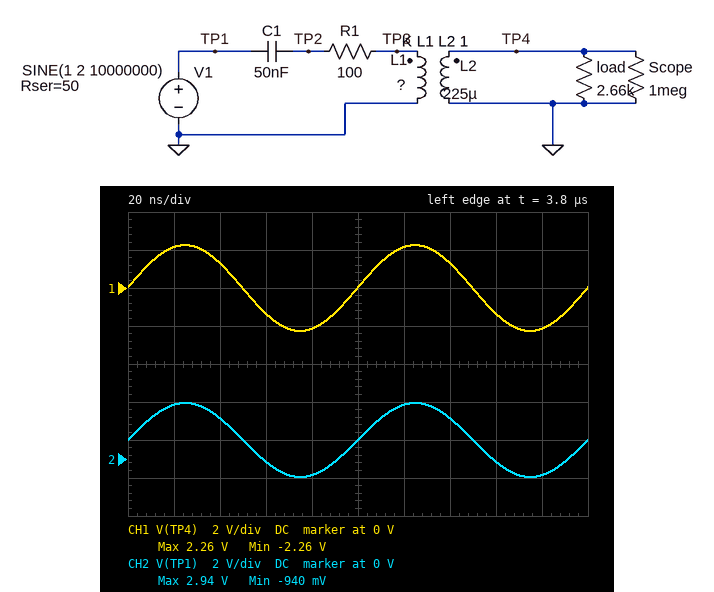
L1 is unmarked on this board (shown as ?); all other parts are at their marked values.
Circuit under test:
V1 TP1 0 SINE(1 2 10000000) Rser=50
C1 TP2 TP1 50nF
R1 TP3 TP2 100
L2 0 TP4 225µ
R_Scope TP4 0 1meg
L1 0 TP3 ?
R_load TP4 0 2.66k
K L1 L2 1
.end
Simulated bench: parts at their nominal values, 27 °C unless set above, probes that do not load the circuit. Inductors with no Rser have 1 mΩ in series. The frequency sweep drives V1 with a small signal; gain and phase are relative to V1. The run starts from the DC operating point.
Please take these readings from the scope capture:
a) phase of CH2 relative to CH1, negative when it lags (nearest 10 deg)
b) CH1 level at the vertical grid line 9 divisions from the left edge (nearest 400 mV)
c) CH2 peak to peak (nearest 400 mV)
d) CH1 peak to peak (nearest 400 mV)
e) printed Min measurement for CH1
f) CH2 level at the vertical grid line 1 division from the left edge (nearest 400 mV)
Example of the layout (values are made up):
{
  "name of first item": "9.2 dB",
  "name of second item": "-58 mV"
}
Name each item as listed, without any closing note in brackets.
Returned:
{
  "phase of CH2 relative to CH1, negative when it lags": "0 deg",
  "CH1 level at the vertical grid line 9 divisions from the left edge": "-2.0 V",
  "CH2 peak to peak": "4.0 V",
  "CH1 peak to peak": "4.4 V",
  "printed Min measurement for CH1": "-2.26 V",
  "CH2 level at the vertical grid line 1 division from the left edge": "2.8 V"
}
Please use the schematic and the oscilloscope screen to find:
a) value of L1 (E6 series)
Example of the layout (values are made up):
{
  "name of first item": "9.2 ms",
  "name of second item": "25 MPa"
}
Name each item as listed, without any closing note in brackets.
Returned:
{
  "value of L1": "150 µH"
}
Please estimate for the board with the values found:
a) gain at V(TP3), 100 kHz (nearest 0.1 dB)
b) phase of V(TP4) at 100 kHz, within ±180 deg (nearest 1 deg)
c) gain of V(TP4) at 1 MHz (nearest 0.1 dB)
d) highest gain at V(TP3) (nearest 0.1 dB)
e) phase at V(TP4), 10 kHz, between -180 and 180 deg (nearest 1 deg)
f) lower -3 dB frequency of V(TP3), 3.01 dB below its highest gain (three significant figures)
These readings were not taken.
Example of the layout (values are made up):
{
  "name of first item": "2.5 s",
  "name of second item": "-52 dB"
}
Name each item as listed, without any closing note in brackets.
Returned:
{
  "gain at V(TP3), 100 kHz": "-5.0 dB",
  "phase of V(TP4) at 100 kHz, within ±180 deg": "65 deg",
  "gain of V(TP4) at 1 MHz": "1.0 dB",
  "highest gain at V(TP3)": "-0.7 dB",
  "phase at V(TP4), 10 kHz, between -180 and 180 deg": "154 deg",
  "lower -3 dB frequency of V(TP3), 3.01 dB below its highest gain": "128 kHz"
}
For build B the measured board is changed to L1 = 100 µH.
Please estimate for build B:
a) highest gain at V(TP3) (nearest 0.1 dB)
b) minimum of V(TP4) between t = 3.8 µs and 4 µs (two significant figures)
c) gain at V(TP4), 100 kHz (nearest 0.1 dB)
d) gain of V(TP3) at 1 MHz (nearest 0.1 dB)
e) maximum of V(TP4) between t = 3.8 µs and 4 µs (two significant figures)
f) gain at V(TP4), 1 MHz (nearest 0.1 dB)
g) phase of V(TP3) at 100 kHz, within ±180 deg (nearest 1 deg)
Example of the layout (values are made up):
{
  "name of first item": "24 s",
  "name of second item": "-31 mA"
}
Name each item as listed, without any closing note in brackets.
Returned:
{
  "highest gain at V(TP3)": "-1.0 dB",
  "minimum of V(TP4) between t = 3.8 µs and 4 µs": "-2.7 V",
  "gain at V(TP4), 100 kHz": "-4.4 dB",
  "gain of V(TP3) at 1 MHz": "-1.2 dB",
  "maximum of V(TP4) between t = 3.8 µs and 4 µs": "2.7 V",
  "gain at V(TP4), 1 MHz": "2.3 dB",
  "phase of V(TP3) at 100 kHz, within ±180 deg": "76 deg"
}
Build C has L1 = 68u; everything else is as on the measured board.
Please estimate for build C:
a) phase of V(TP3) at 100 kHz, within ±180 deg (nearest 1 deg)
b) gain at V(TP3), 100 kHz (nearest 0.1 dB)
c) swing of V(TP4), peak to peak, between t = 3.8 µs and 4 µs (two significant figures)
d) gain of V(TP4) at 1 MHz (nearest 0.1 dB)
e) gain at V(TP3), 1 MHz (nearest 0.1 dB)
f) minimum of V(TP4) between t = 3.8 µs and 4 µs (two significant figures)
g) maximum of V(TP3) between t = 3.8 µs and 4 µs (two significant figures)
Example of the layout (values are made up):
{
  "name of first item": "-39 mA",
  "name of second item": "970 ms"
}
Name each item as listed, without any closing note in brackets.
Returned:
{
  "phase of V(TP3) at 100 kHz, within ±180 deg": "83 deg",
  "gain at V(TP3), 100 kHz": "-11.1 dB",
  "swing of V(TP4), peak to peak, between t = 3.8 µs and 4 µs": "6.1 V",
  "gain of V(TP4) at 1 MHz": "3.4 dB",
  "gain at V(TP3), 1 MHz": "-1.8 dB",
  "minimum of V(TP4) between t = 3.8 µs and 4 µs": "-3.1 V",
  "maximum of V(TP3) between t = 3.8 µs and 4 µs": "1.7 V"
}
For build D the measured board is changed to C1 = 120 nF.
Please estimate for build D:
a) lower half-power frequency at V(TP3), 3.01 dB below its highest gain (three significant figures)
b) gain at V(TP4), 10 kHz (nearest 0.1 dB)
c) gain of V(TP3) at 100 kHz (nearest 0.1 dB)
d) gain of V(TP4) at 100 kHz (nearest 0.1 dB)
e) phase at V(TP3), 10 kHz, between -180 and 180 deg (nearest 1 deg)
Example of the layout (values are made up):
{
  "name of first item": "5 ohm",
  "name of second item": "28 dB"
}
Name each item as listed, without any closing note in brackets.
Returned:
{
  "lower half-power frequency at V(TP3), 3.01 dB below its highest gain": "139 kHz",
  "gain at V(TP4), 10 kHz": "-24.5 dB",
  "gain of V(TP3) at 100 kHz": "-5.4 dB",
  "gain of V(TP4) at 100 kHz": "-3.6 dB",
  "phase at V(TP3), 10 kHz, between -180 and 180 deg": "129 deg"
}
